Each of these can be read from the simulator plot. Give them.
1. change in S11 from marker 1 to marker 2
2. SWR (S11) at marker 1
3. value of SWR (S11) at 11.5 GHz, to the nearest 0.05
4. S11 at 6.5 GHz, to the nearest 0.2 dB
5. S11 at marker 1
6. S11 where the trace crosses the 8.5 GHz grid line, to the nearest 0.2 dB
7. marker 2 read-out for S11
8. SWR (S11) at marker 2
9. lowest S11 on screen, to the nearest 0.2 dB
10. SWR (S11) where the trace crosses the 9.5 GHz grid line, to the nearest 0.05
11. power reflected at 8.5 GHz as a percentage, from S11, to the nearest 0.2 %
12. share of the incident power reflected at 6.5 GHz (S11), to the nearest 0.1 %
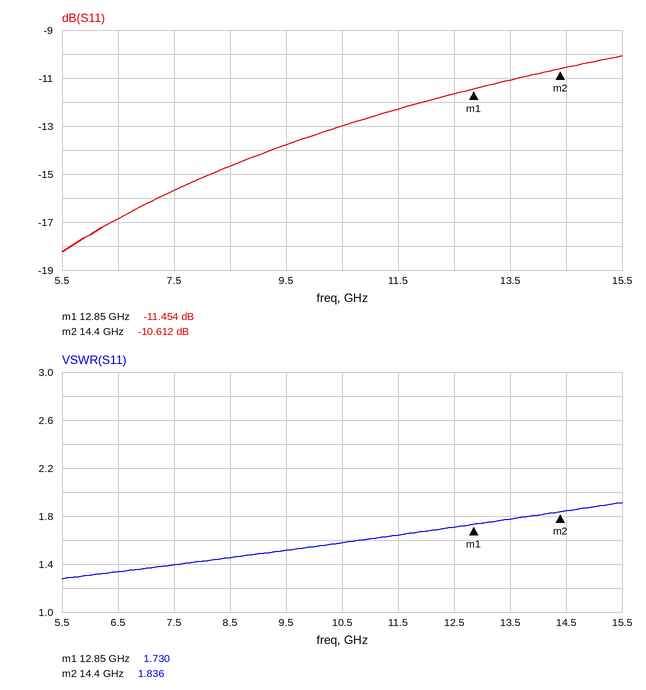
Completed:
0.842 dB
1.730
1.65
-16.8 dB
-11.454 dB
-14.6 dB
-10.612 dB
1.836
-18.2 dB
1.50
3.4 %
2.1 %
